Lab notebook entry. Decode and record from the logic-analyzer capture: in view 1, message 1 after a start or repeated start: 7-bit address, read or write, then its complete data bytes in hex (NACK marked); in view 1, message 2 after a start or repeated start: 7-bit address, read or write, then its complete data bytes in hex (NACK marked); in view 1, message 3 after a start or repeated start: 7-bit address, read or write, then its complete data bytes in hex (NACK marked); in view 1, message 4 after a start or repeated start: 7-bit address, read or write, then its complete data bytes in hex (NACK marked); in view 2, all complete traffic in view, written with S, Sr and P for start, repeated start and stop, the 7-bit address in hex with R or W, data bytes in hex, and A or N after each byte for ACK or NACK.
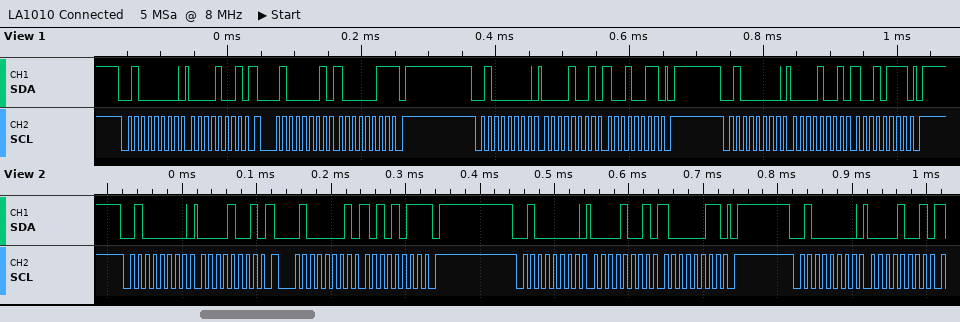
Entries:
0x20 write: 09
0x20 read: 83 NACK
0x20 write: 09 93
0x20 write: 09 97
S 20W A 09 A Sr 20R A AB N P S 20W A 09 A 83 A P S 20W A 09 A
